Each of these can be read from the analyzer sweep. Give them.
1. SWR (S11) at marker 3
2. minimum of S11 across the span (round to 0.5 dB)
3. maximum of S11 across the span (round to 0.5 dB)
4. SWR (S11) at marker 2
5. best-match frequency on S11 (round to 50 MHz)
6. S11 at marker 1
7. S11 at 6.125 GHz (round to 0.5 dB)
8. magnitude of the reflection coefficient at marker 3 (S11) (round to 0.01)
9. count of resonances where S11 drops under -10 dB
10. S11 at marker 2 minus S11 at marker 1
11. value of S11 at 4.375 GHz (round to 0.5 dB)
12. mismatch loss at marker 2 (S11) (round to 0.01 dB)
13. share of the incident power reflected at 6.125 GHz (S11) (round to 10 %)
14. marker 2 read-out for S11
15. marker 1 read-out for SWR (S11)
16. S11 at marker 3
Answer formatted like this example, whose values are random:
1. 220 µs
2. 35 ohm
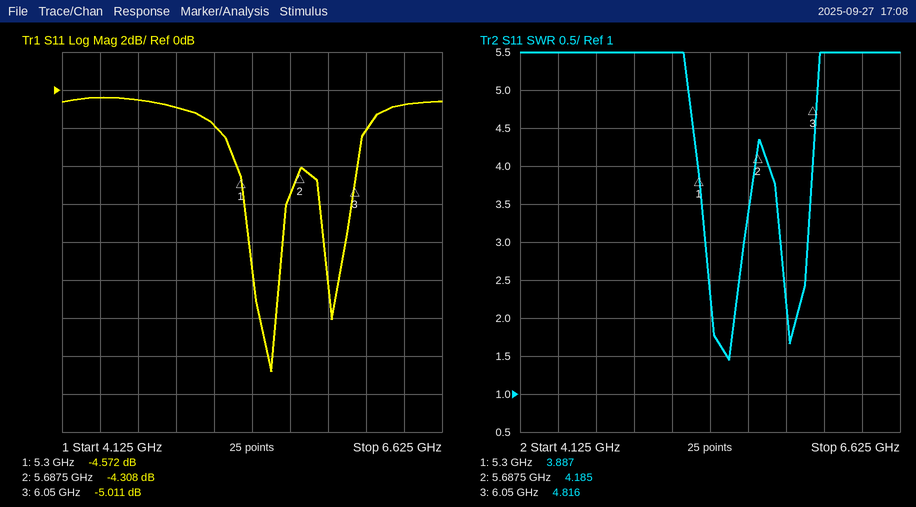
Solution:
1. 4.816
2. -15.0 dB
3. -0.5 dB
4. 4.185
5. 5.50 GHz
6. -4.572 dB
7. -2.0 dB
8. 0.56
9. 2
10. 0.264 dB
11. -0.5 dB
12. 2.01 dB
13. 60 %
14. -4.308 dB
15. 3.887
16. -5.011 dB
